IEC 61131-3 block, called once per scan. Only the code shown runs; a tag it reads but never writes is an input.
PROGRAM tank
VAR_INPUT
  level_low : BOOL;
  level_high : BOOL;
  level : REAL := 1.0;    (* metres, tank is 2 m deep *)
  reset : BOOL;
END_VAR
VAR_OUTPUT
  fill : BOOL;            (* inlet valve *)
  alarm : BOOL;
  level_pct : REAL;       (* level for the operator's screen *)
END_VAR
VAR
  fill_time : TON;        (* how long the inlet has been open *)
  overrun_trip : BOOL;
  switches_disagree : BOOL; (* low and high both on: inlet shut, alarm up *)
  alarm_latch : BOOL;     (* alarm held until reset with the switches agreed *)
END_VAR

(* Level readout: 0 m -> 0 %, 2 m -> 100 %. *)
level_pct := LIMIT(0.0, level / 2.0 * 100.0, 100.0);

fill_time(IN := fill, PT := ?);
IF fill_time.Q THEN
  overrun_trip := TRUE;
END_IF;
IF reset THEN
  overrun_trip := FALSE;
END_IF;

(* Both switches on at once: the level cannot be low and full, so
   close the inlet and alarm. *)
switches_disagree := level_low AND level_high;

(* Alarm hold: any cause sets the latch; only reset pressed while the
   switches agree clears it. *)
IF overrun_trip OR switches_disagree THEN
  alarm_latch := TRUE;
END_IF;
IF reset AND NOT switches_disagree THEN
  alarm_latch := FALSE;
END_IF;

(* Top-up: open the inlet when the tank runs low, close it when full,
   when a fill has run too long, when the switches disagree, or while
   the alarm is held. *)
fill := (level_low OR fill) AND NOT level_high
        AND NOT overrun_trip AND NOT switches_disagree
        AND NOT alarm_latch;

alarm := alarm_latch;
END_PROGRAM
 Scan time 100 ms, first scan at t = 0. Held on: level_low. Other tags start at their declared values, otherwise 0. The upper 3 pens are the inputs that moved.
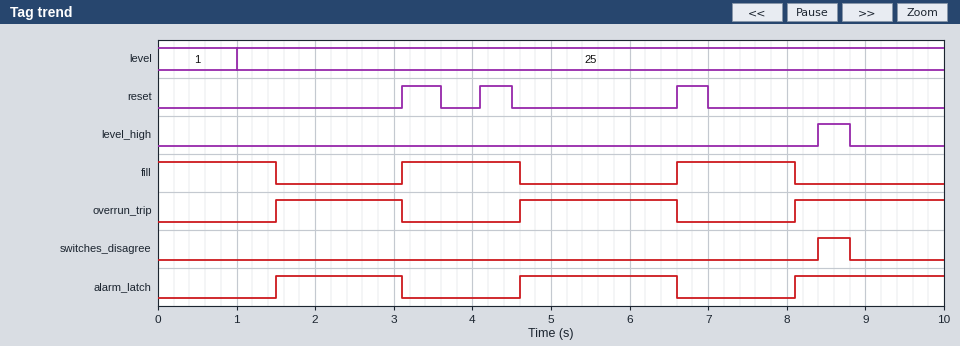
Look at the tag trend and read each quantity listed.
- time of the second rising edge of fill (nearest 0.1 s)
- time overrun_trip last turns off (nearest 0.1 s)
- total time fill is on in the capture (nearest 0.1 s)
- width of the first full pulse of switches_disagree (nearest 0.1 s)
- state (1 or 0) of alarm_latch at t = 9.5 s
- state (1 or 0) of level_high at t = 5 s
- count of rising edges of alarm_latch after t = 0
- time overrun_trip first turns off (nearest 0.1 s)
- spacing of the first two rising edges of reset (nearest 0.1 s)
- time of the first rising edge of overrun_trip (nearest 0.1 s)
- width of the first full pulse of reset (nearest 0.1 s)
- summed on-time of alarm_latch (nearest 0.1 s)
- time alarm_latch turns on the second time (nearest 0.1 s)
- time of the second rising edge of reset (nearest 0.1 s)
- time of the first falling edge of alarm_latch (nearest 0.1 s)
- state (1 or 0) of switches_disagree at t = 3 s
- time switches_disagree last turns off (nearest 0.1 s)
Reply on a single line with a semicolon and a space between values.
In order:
6.6 s; 6.6 s; 4.5 s; 0.4 s; 1; 0; 3; 3.1 s; 1.0 s; 1.5 s; 0.5 s; 5.5 s; 4.6 s; 4.1 s; 3.1 s; 0; 8.8 s
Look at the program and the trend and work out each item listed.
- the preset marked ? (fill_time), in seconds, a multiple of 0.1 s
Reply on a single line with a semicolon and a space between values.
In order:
1.4 s
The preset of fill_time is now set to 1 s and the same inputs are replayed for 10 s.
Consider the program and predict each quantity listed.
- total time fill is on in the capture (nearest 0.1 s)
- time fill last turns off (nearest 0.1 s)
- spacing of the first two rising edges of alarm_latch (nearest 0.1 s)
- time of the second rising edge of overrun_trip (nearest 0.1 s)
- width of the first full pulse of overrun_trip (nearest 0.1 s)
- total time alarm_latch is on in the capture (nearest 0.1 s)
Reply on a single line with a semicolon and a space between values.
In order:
3.6 s; 7.7 s; 3.4 s; 4.5 s; 2.0 s; 6.4 s
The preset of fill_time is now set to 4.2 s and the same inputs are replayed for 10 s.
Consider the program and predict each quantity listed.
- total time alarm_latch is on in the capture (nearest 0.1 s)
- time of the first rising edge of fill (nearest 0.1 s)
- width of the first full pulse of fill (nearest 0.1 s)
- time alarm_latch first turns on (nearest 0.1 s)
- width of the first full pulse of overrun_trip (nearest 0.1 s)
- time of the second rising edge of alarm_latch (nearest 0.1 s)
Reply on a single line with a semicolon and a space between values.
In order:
3.7 s; 6.6 s; 1.8 s; 4.5 s; 2.1 s; 8.4 s
